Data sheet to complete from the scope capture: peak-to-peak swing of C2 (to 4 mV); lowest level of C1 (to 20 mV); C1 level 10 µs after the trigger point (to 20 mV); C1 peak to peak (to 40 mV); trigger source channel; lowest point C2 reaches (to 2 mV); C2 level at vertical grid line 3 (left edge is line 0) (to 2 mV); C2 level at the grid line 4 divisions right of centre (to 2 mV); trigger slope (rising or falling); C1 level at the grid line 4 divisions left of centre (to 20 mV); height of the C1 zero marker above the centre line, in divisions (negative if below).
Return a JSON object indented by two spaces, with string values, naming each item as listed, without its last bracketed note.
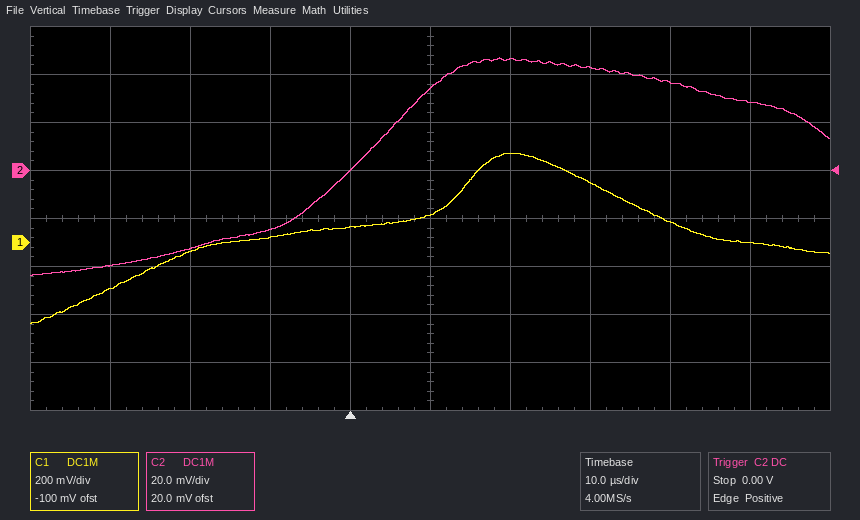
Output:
{
  "peak-to-peak swing of C2": "92 mV",
  "lowest level of C1": "-340 mV",
  "C1 level 10 µs after the trigger point": "120 mV",
  "C1 peak to peak": "720 mV",
  "trigger source channel": "C2",
  "lowest point C2 reaches": "-44 mV",
  "C2 level at vertical grid line 3 (left edge is line 0)": "-24 mV",
  "C2 level at the grid line 4 divisions right of centre": "28 mV",
  "trigger slope": "rising",
  "C1 level at the grid line 4 divisions left of centre": "-200 mV",
  "height of the C1 zero marker above the centre line, in divisions": "-0.5 div"
}
